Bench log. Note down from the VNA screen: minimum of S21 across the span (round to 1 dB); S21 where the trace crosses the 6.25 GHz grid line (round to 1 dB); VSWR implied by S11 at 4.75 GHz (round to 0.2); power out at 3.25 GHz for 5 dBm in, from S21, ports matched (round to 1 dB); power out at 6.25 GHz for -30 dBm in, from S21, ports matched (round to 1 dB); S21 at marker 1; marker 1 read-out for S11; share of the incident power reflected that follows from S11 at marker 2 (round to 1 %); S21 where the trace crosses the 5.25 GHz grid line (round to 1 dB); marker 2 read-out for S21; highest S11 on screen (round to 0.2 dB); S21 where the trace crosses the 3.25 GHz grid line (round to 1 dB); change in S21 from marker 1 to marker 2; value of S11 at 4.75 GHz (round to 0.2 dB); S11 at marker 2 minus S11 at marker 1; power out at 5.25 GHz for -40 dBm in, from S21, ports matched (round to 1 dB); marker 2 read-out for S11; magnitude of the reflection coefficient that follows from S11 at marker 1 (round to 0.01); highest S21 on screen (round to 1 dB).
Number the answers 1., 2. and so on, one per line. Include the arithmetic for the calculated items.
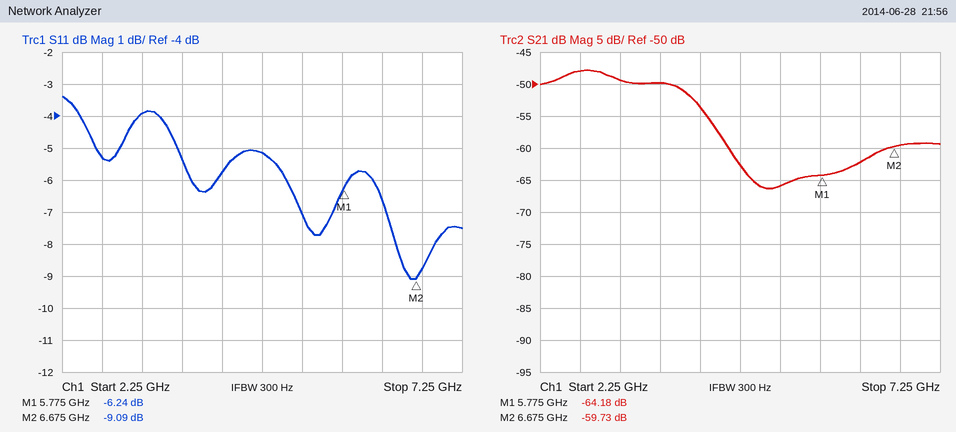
1. -66 dB
2. -62 dB
3. |Γ| = 10^(-5.2/20) = 0.5495; VSWR = (1 + 0.5495)/(1 − 0.5495) ≈ 3.4
4. 5 dBm + (-49 dB) = -44 dBm
5. -30 dBm + (-62 dB) = -92 dBm
6. -64.18 dB
7. -6.24 dB
8. 10^(-9.09/10) ≈ 12 %
9. -66 dB
10. -59.73 dB
11. -3.4 dB
12. -49 dB
13. -59.73 − (-64.18) = 4.45 dB
14. -5.2 dB
15. -9.09 − (-6.24) = -2.85 dB
16. -40 dBm + (-66 dB) = -106 dBm
17. -9.09 dB
18. 10^(-6.24/20) ≈ 0.49
19. -48 dB
